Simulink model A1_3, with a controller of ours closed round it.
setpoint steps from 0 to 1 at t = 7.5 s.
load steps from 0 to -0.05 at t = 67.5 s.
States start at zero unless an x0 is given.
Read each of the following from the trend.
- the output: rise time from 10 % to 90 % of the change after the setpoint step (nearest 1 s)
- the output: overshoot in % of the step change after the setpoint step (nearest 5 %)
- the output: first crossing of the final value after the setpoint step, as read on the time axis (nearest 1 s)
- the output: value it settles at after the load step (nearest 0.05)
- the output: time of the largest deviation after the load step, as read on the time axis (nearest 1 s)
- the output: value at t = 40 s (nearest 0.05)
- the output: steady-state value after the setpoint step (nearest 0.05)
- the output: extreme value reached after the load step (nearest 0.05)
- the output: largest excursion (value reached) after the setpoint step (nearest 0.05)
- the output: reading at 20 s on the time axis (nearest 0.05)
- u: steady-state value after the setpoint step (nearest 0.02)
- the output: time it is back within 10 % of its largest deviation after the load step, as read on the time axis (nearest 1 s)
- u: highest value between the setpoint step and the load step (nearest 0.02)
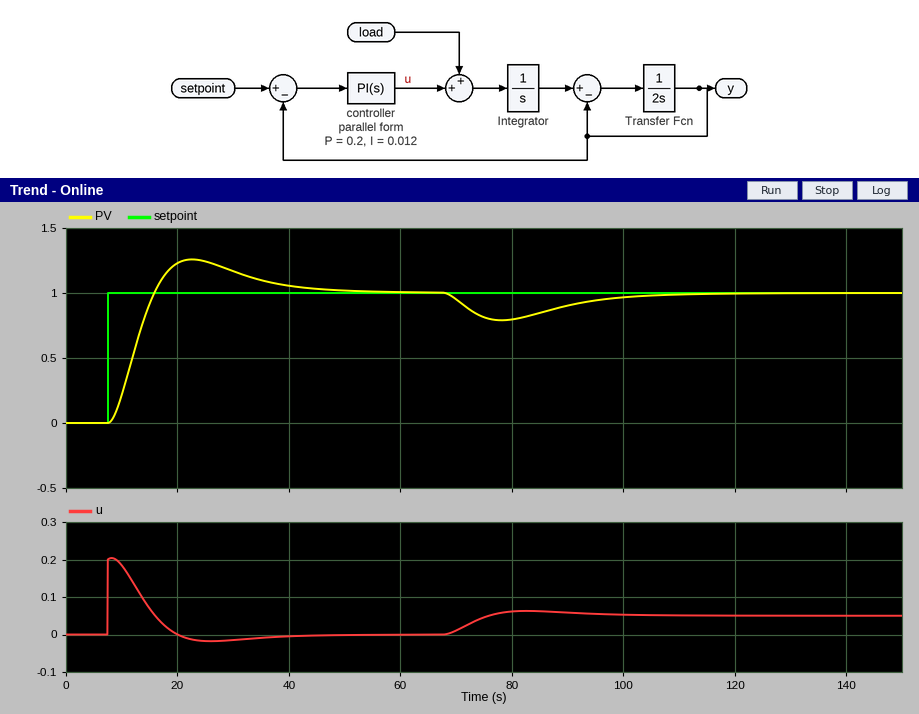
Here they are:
6 s
25 %
16 s
1.00
78 s
1.05
1.00
0.80
1.25
1.25
0.00
104 s
0.20
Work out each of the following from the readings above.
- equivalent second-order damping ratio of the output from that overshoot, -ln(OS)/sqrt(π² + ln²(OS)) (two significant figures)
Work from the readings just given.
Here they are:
0.40
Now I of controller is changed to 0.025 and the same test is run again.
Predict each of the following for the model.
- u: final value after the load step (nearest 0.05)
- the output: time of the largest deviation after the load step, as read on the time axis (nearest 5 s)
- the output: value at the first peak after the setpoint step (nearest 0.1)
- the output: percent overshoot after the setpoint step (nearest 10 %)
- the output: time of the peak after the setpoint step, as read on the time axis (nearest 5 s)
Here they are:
0.05
75 s
1.4
40 %
20 s
